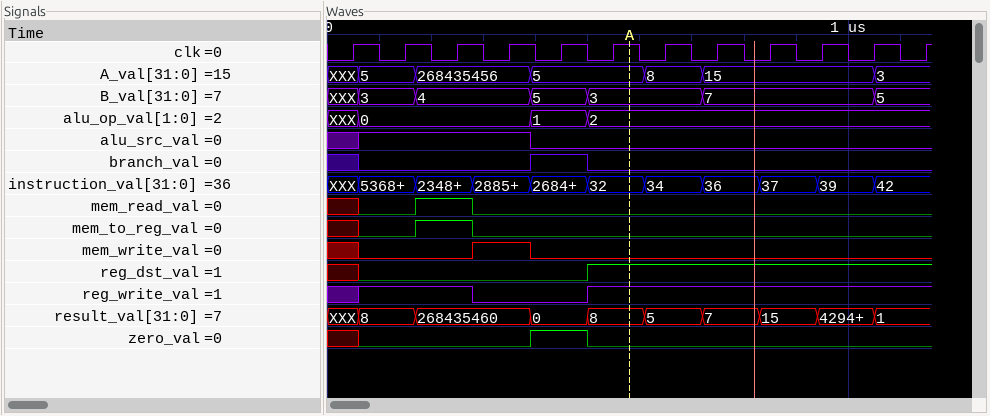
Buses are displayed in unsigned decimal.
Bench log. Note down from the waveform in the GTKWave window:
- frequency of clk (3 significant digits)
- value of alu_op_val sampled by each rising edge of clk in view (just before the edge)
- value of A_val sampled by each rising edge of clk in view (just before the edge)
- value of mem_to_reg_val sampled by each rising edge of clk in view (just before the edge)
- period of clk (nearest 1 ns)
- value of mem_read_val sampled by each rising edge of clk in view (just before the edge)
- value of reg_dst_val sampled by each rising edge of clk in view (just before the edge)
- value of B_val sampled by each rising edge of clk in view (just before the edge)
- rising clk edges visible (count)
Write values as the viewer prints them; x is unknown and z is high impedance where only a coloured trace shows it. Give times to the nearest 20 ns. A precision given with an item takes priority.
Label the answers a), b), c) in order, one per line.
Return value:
a) 10.0 MHz
b) XXX, 0, 0, 0, 1, 2, 2, 2, 2, 2, 2, 2
c) XXX, 5, 268435456, 268435456, 5, 5, 8, 15, 15, 15, 15, 3
d) x 0 1 0 0 0 0 0 0 0 0 0
e) 100 ns
f) x 0 1 0 0 0 0 0 0 0 0 0
g) x 0 0 0 0 1 1 1 1 1 1 1
h) XXX, 3, 4, 4, 5, 3, 3, 7, 7, 7, 7, 5
i) 12
